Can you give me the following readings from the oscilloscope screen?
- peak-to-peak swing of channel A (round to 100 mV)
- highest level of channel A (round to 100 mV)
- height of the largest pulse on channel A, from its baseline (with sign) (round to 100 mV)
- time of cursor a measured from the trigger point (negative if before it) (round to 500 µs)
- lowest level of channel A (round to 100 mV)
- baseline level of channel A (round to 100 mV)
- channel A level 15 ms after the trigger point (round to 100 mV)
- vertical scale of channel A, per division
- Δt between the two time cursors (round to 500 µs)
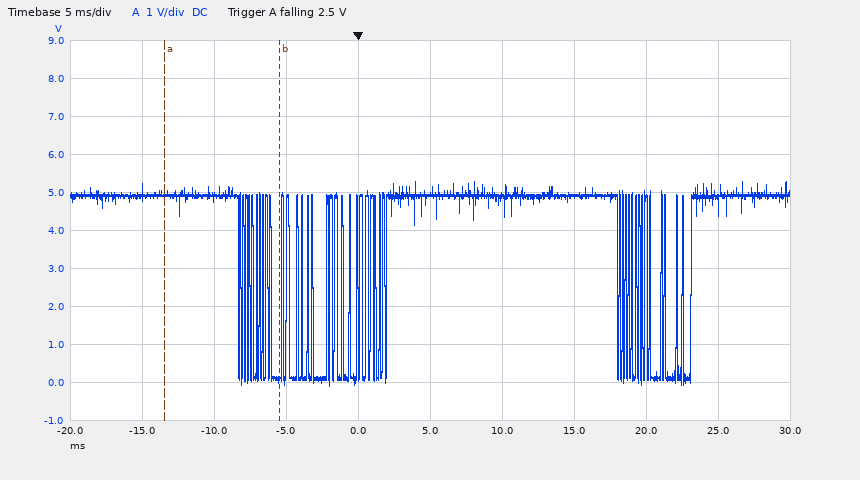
5.4 V
5.3 V
-5.0 V
-13.5 ms
-100 mV
4.9 V
4.9 V
1 V
8.0 ms
